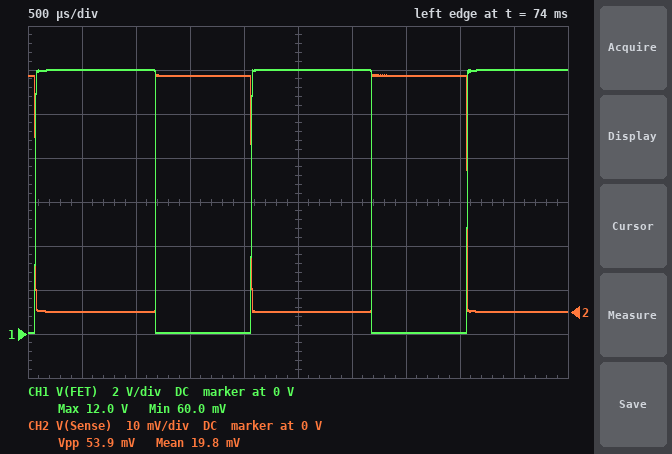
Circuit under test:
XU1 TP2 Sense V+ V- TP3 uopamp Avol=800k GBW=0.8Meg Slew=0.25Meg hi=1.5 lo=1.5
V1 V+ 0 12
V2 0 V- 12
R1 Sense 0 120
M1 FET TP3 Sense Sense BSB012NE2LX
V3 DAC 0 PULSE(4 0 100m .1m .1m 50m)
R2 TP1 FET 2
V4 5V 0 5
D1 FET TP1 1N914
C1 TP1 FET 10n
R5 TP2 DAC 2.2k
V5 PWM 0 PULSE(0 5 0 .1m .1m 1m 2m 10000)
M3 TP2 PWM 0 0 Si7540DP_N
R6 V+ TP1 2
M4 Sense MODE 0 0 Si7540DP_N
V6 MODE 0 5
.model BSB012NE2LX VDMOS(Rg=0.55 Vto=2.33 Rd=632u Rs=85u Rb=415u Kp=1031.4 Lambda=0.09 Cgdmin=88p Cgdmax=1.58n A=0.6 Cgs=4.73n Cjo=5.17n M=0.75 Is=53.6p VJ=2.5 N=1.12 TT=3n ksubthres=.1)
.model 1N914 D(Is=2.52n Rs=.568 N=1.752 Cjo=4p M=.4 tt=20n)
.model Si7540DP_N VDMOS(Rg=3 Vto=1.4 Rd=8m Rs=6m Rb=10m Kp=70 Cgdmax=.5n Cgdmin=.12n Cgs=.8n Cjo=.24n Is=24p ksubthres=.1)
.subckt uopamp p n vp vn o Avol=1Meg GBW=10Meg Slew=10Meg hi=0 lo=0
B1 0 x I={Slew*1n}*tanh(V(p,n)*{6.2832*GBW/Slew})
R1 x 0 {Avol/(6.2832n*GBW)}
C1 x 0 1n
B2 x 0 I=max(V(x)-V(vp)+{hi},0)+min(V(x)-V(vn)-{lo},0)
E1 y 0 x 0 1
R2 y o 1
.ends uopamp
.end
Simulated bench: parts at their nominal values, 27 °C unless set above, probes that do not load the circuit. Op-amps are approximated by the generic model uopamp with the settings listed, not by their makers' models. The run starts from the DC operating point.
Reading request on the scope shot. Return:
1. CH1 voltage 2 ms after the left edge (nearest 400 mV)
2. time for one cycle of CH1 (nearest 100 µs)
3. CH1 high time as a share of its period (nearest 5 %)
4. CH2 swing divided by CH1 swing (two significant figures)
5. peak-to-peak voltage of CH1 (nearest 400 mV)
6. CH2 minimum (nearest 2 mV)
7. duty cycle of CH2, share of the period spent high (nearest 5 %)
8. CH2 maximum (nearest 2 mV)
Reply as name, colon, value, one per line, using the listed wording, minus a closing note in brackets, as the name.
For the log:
CH1 voltage 2 ms after the left edge: 0 V
time for one cycle of CH1: 2.0 ms
CH1 high time as a share of its period: 55 %
CH2 swing divided by CH1 swing: 0.0045
peak-to-peak voltage of CH1: 12.0 V
CH2 minimum: 0 V
duty cycle of CH2, share of the period spent high: 45 %
CH2 maximum: 54 mV
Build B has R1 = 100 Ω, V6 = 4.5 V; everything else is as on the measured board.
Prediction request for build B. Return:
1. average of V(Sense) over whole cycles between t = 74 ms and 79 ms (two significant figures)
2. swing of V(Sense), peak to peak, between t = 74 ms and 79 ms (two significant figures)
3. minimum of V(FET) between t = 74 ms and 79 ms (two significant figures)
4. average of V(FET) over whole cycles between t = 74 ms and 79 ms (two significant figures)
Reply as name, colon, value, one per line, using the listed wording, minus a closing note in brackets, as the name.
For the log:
average of V(Sense) over whole cycles between t = 74 ms and 79 ms: 25 mV
swing of V(Sense), peak to peak, between t = 74 ms and 79 ms: 56 mV
minimum of V(FET) between t = 74 ms and 79 ms: 58 mV
average of V(FET) over whole cycles between t = 74 ms and 79 ms: 6.7 V
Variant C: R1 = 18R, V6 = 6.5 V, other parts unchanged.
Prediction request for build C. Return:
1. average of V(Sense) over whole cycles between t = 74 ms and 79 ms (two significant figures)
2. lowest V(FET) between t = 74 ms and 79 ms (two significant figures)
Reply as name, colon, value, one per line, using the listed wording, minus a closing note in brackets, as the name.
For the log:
average of V(Sense) over whole cycles between t = 74 ms and 79 ms: 22 mV
lowest V(FET) between t = 74 ms and 79 ms: 53 mV
